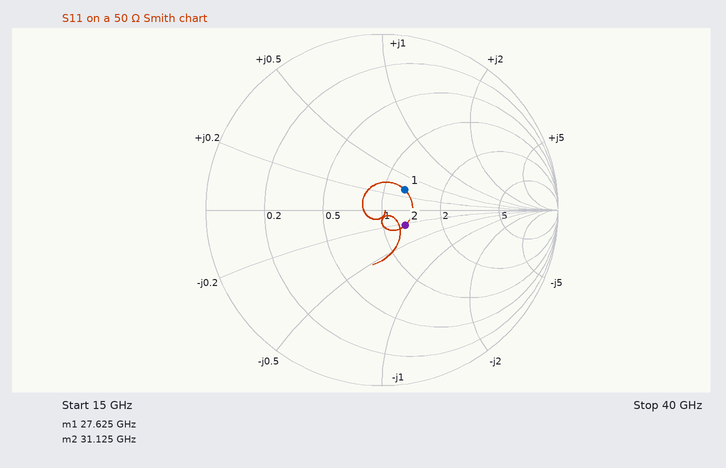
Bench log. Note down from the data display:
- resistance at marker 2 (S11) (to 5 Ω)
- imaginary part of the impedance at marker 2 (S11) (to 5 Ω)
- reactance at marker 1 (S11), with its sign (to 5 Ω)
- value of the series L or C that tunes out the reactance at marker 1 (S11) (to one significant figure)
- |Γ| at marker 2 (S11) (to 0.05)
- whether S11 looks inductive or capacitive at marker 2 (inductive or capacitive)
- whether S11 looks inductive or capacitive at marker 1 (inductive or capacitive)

65 Ω
-10 Ω
+15 Ω
400 fF
0.15
capacitive
inductive
